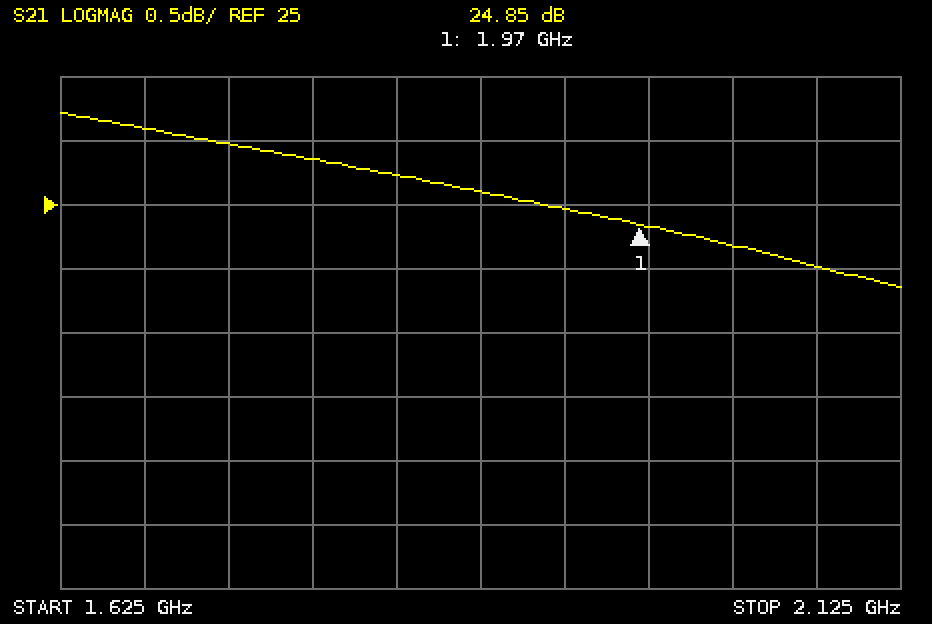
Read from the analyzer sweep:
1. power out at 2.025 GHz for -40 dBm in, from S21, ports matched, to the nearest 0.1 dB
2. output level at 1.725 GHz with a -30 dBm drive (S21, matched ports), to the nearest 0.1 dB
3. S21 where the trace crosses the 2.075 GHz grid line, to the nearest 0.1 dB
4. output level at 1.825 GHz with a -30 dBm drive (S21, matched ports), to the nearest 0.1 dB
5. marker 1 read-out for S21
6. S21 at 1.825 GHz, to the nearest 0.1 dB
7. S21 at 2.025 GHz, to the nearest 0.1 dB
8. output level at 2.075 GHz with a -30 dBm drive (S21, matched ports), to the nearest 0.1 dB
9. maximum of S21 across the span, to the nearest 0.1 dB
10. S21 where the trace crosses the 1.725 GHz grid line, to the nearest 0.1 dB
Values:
-15.3 dBm
-4.5 dBm
24.5 dB
-4.8 dBm
24.85 dB
25.2 dB
24.7 dB
-5.5 dBm
25.7 dB
25.5 dB
